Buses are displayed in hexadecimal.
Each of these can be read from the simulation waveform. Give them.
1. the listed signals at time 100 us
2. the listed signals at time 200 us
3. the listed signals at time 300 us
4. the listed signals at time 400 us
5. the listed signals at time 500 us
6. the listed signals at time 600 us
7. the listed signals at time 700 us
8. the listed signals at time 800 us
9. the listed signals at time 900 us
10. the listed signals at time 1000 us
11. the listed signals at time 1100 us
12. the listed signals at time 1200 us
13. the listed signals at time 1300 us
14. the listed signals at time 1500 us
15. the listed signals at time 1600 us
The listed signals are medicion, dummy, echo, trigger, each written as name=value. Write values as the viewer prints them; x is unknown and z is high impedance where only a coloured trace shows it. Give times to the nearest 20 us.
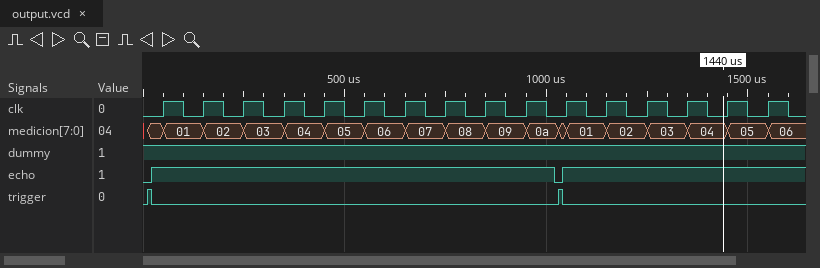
medicion=01, dummy=1, echo=1, trigger=0
medicion=02, dummy=1, echo=1, trigger=0
medicion=03, dummy=1, echo=1, trigger=0
medicion=04, dummy=1, echo=1, trigger=0
medicion=05, dummy=1, echo=1, trigger=0
medicion=06, dummy=1, echo=1, trigger=0
medicion=07, dummy=1, echo=1, trigger=0
medicion=08, dummy=1, echo=1, trigger=0
medicion=09, dummy=1, echo=1, trigger=0
medicion=0a, dummy=1, echo=1, trigger=0
medicion=01, dummy=1, echo=1, trigger=0
medicion=02, dummy=1, echo=1, trigger=0
medicion=03, dummy=1, echo=1, trigger=0
medicion=05, dummy=1, echo=1, trigger=0
medicion=06, dummy=1, echo=1, trigger=0
